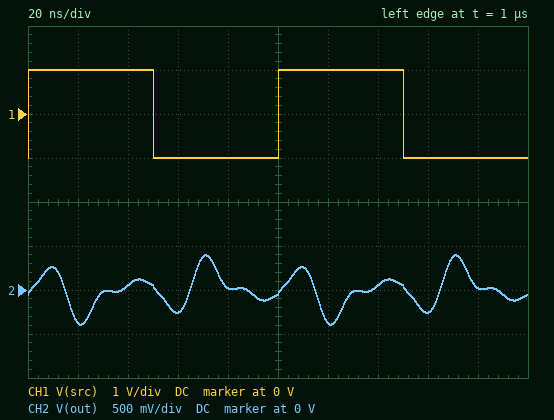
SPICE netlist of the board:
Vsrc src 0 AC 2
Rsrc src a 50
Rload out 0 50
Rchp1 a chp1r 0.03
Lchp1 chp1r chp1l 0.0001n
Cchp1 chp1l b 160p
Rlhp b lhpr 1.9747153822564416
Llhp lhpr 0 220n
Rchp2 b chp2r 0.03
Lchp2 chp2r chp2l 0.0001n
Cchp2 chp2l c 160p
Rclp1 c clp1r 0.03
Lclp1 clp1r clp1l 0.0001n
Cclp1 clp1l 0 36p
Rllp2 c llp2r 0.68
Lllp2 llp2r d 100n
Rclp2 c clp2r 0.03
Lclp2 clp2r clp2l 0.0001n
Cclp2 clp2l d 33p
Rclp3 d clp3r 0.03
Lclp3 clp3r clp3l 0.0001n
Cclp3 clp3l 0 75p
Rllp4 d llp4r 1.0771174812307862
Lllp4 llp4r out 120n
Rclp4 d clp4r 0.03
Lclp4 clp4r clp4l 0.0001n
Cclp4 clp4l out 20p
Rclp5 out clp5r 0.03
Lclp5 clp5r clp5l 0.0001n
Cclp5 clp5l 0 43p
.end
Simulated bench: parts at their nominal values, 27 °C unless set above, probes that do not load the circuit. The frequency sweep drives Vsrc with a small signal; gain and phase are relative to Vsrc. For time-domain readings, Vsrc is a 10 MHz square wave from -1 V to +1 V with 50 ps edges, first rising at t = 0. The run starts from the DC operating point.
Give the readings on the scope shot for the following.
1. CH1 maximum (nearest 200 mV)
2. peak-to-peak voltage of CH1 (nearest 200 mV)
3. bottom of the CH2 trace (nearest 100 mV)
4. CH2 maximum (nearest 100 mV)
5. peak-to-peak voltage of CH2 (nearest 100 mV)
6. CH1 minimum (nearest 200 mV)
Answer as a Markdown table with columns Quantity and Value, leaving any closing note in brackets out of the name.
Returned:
| Quantity | Value |
|---|---|
| CH1 maximum | 1.0 V |
| peak-to-peak voltage of CH1 | 2.0 V |
| bottom of the CH2 trace | -400 mV |
| CH2 maximum | 400 mV |
| peak-to-peak voltage of CH2 | 800 mV |
| CH1 minimum | -1.0 V |
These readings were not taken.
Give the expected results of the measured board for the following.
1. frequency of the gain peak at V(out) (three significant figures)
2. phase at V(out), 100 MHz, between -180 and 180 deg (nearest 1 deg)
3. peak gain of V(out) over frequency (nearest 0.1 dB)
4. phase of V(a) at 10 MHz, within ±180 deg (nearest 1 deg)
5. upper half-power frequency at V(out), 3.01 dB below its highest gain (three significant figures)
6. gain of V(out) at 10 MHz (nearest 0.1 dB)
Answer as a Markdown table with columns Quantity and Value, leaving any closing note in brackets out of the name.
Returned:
| Quantity | Value |
|---|---|
| frequency of the gain peak at V(out) | 42.5 MHz |
| phase at V(out), 100 MHz, between -180 and 180 deg | -160 deg |
| peak gain of V(out) over frequency | -6.5 dB |
| phase of V(a) at 10 MHz, within ±180 deg | -30 deg |
| upper half-power frequency at V(out), 3.01 dB below its highest gain | 67.5 MHz |
| gain of V(out) at 10 MHz | -24.1 dB |
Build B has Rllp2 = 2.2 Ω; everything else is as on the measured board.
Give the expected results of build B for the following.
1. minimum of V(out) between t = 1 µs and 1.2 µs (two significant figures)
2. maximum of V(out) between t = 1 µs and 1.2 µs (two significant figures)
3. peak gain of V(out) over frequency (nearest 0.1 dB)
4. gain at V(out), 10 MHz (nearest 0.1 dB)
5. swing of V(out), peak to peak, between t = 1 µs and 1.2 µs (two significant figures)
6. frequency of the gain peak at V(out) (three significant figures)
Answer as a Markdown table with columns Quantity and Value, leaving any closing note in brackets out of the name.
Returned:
| Quantity | Value |
|---|---|
| minimum of V(out) between t = 1 µs and 1.2 µs | -380 mV |
| maximum of V(out) between t = 1 µs and 1.2 µs | 380 mV |
| peak gain of V(out) over frequency | -6.8 dB |
| gain at V(out), 10 MHz | -24.2 dB |
| swing of V(out), peak to peak, between t = 1 µs and 1.2 µs | 760 mV |
| frequency of the gain peak at V(out) | 38.3 MHz |
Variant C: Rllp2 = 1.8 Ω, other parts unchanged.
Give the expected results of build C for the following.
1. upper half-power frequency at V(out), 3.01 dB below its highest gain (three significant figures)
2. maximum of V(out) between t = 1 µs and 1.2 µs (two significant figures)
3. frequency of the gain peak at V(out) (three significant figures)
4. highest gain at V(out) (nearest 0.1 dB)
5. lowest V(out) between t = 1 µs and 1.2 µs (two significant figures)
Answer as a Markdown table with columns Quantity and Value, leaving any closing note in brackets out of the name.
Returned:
| Quantity | Value |
|---|---|
| upper half-power frequency at V(out), 3.01 dB below its highest gain | 66.9 MHz |
| maximum of V(out) between t = 1 µs and 1.2 µs | 380 mV |
| frequency of the gain peak at V(out) | 39.2 MHz |
| highest gain at V(out) | -6.7 dB |
| lowest V(out) between t = 1 µs and 1.2 µs | -380 mV |
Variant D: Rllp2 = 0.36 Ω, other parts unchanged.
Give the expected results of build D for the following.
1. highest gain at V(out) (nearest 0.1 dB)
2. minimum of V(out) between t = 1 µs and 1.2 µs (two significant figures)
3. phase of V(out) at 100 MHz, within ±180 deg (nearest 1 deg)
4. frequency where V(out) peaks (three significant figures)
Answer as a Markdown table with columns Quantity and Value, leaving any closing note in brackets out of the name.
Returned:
| Quantity | Value |
|---|---|
| highest gain at V(out) | -6.4 dB |
| minimum of V(out) between t = 1 µs and 1.2 µs | -400 mV |
| phase of V(out) at 100 MHz, within ±180 deg | -159 deg |
| frequency where V(out) peaks | 43.5 MHz |
